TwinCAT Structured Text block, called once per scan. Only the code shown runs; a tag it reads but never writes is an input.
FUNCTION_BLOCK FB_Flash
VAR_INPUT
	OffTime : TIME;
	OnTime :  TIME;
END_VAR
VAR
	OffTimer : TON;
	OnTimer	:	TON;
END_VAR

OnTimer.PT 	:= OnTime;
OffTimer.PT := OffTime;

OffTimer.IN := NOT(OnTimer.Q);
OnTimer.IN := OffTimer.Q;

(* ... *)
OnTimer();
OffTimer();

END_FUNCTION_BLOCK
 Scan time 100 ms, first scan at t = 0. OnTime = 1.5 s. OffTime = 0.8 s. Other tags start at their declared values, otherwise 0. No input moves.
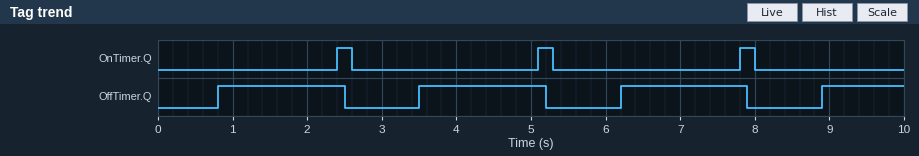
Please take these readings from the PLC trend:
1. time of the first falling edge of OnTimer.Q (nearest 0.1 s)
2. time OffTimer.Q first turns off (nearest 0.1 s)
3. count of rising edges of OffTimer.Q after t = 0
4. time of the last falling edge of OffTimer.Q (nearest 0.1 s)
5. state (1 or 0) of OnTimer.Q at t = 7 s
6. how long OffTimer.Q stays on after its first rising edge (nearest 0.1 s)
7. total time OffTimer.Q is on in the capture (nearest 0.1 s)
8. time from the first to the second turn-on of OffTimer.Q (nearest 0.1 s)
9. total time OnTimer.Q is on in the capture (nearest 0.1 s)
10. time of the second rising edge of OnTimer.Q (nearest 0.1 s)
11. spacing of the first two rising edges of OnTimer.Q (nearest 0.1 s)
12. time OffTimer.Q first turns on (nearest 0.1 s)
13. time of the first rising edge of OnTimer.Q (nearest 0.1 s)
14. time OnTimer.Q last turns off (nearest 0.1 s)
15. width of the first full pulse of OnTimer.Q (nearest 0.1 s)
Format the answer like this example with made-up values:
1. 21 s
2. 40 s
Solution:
1. 2.6 s
2. 2.5 s
3. 4
4. 7.9 s
5. 0
6. 1.7 s
7. 6.2 s
8. 2.7 s
9. 0.6 s
10. 5.1 s
11. 2.7 s
12. 0.8 s
13. 2.4 s
14. 8.0 s
15. 0.2 s
